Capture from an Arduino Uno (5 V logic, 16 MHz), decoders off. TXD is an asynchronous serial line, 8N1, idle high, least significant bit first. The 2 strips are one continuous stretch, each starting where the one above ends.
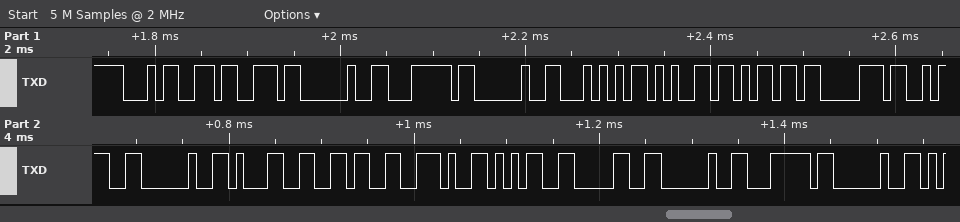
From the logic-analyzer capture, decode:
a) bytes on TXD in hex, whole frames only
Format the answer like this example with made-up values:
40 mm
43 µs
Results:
0x34 0x73 0x20 0x7C 0x20 0x54 0x65 0x6D 0x70 0x3A 0x20 0x31 0x36 0x2E 0x35 0x30 0x20 0x7C 0x20
